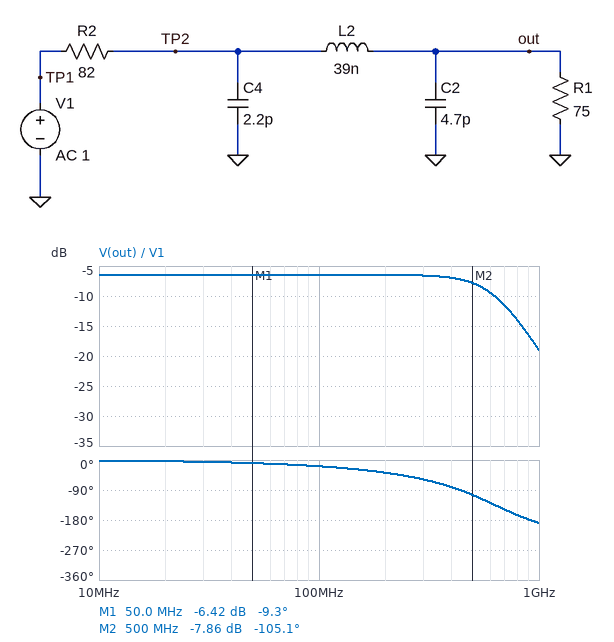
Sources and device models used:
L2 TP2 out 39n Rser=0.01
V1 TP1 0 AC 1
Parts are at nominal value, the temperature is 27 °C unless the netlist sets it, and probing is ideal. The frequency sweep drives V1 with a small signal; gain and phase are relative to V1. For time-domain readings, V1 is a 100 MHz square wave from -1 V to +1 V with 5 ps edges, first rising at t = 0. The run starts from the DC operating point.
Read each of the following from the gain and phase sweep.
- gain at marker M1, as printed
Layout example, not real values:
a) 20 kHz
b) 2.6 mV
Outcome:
a) -6.42 dB
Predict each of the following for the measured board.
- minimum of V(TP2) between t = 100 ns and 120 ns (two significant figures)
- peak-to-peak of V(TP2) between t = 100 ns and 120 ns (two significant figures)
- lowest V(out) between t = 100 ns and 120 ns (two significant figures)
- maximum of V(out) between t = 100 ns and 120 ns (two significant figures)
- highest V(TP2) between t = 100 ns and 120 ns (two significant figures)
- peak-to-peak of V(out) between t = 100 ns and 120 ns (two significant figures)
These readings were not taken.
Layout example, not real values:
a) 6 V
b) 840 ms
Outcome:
a) -900 mV
b) 1.8 V
c) -540 mV
d) 540 mV
e) 900 mV
f) 1.1 V
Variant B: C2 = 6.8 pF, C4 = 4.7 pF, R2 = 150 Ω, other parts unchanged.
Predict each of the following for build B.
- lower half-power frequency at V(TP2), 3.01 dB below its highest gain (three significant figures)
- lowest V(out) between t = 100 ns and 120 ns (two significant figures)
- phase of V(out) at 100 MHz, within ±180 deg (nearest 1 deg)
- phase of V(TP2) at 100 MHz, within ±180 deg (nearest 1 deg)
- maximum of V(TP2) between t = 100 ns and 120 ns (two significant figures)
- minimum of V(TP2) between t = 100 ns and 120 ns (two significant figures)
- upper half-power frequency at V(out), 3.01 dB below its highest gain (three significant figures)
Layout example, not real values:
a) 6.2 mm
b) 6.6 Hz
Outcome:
a) 381 MHz
b) -400 mV
c) -26 deg
d) -6 deg
e) 500 mV
f) -500 mV
g) 529 MHz
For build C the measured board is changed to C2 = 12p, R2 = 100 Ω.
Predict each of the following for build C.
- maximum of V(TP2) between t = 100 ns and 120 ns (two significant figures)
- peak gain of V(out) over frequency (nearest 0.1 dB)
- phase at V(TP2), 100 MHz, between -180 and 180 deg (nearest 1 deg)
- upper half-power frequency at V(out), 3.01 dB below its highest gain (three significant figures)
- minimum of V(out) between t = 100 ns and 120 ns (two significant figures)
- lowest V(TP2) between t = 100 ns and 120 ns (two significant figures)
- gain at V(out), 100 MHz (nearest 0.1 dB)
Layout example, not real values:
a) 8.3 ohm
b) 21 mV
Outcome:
a) 830 mV
b) -7.4 dB
c) -8 deg
d) 367 MHz
e) -430 mV
f) -830 mV
g) -7.7 dB
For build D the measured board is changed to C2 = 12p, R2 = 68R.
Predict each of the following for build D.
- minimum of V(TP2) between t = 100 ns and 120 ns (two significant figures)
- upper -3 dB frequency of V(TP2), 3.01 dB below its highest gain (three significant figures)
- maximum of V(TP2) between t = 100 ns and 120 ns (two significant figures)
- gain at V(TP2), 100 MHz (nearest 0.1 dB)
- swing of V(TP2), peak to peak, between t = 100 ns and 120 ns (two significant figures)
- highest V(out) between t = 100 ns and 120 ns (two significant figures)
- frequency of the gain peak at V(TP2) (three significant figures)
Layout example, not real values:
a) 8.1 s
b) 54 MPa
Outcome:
a) -940 mV
b) 1.34 GHz
c) 940 mV
d) -6.8 dB
e) 1.9 V
f) 570 mV
g) 624 MHz
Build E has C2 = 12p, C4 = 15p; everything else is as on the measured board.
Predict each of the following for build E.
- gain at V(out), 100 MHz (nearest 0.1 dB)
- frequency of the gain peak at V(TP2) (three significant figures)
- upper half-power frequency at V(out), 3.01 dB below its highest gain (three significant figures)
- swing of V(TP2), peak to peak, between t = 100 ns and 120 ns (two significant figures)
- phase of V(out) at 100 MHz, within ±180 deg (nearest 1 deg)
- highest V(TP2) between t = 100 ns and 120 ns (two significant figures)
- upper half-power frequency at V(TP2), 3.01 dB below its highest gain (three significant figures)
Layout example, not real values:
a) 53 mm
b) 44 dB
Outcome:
a) -7.2 dB
b) 322 MHz
c) 340 MHz
d) 1.0 V
e) -44 deg
f) 520 mV
g) 432 MHz
